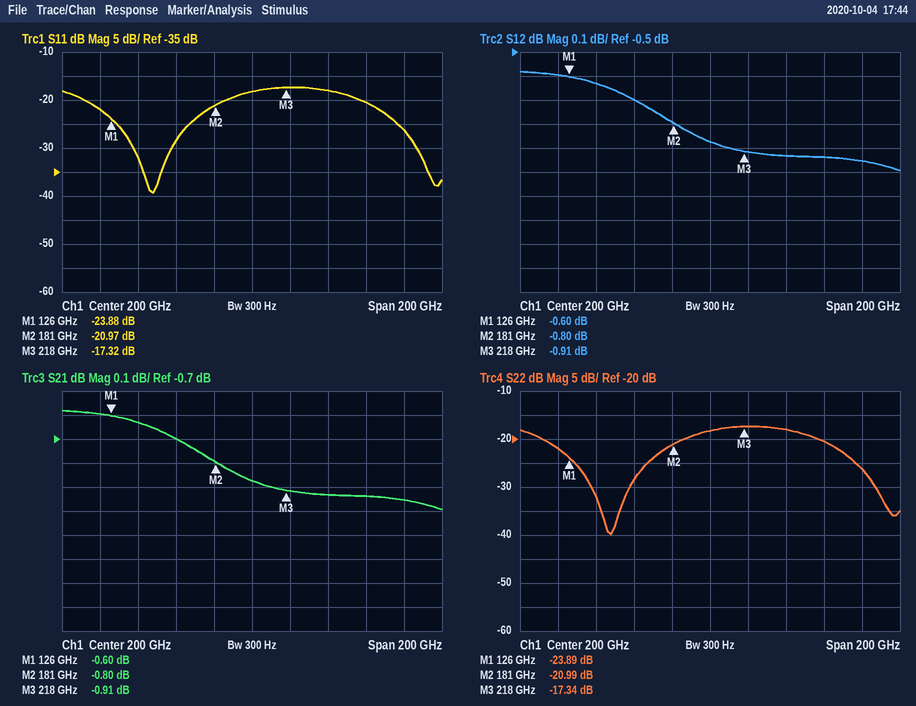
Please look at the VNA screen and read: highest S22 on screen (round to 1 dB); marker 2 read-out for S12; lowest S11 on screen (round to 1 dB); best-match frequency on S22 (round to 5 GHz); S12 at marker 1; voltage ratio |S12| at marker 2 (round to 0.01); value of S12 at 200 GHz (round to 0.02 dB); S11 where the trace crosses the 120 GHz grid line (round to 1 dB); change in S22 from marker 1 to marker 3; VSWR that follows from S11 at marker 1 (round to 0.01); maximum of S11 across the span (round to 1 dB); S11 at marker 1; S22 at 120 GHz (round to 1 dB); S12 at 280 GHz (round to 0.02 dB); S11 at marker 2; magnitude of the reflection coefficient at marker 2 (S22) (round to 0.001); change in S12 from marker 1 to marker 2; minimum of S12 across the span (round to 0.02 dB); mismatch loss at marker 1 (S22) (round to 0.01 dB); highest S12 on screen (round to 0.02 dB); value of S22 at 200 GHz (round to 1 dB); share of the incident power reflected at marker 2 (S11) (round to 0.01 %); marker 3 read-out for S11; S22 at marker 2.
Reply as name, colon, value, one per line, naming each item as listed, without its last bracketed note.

highest S22 on screen: -17 dB
marker 2 read-out for S12: -0.80 dB
lowest S11 on screen: -39 dB
best-match frequency on S22: 150 GHz
S12 at marker 1: -0.60 dB
voltage ratio |S12| at marker 2: 0.91
value of S12 at 200 GHz: -0.88 dB
S11 where the trace crosses the 120 GHz grid line: -22 dB
change in S22 from marker 1 to marker 3: 6.55 dB
VSWR that follows from S11 at marker 1: 1.14
maximum of S11 across the span: -17 dB
S11 at marker 1: -23.88 dB
S22 at 120 GHz: -22 dB
S12 at 280 GHz: -0.96 dB
S11 at marker 2: -20.97 dB
magnitude of the reflection coefficient at marker 2 (S22): 0.089
change in S12 from marker 1 to marker 2: -0.20 dB
minimum of S12 across the span: -1.00 dB
mismatch loss at marker 1 (S22): 0.02 dB
highest S12 on screen: -0.58 dB
value of S22 at 200 GHz: -18 dB
share of the incident power reflected at marker 2 (S11): 0.80 %
marker 3 read-out for S11: -17.32 dB
S22 at marker 2: -20.99 dB
